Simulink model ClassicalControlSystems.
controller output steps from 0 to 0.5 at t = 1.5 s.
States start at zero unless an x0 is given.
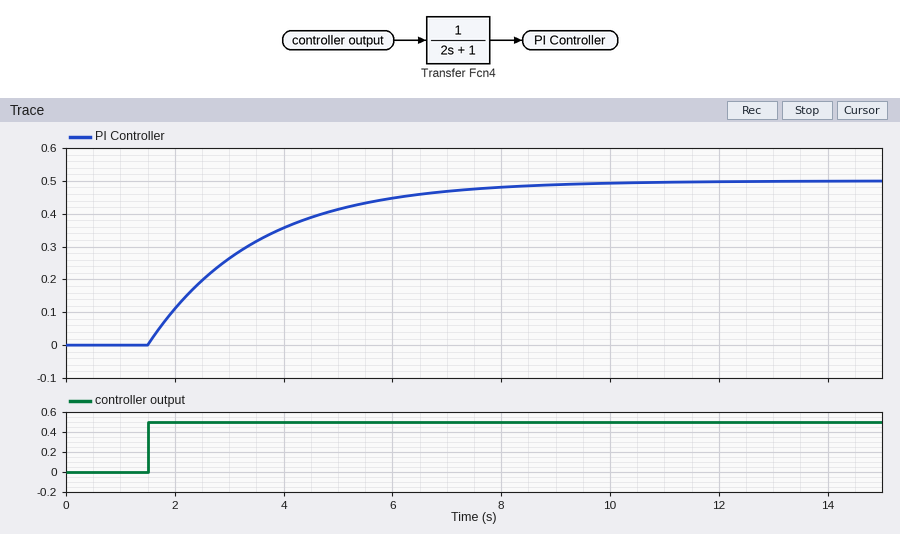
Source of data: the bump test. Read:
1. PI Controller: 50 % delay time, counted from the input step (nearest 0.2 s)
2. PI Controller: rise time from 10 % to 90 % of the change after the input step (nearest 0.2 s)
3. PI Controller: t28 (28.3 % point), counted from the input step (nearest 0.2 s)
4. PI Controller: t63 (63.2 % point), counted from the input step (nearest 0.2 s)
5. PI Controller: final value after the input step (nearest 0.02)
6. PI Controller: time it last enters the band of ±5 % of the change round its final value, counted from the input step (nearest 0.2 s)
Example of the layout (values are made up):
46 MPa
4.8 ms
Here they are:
1.4 s
4.4 s
0.6 s
2.0 s
0.50
6.0 s
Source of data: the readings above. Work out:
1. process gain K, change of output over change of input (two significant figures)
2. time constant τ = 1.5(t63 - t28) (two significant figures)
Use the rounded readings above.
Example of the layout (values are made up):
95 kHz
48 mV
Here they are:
1.0
2.1 s
